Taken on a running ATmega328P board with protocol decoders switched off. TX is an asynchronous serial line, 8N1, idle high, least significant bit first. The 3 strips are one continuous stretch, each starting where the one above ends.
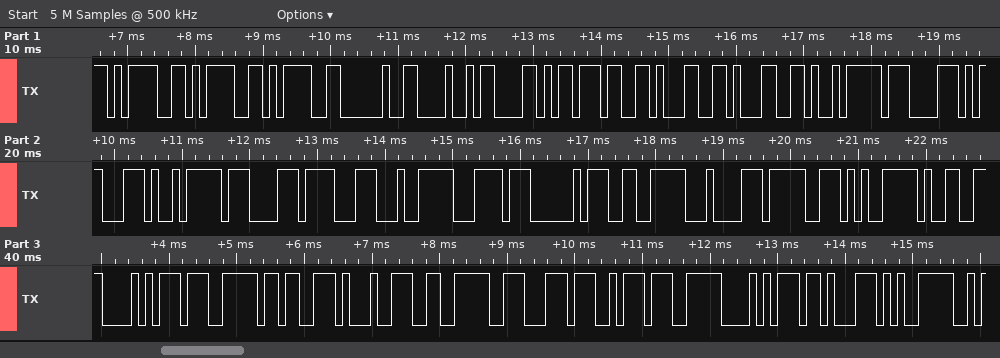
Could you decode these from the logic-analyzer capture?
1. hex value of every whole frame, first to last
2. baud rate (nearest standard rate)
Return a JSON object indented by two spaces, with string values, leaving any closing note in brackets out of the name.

{
  "hex value of every whole frame, first to last": "0x3D 0x3D 0x3D 0x20 0x48 0x58 0x37 0x31 0x31 0xE9 0x87 0x8D 0xE9 0x87 0x8F 0xE4 0xBC 0xA0 0xE6 0x84 0x9F 0xE5 0x99 0xA8 0xE7 0x9B 0x91 0xE6 0x8E 0xA7 0xE7 0xA8 0x8B 0xE5",
  "baud rate": "9600 baud"
}
